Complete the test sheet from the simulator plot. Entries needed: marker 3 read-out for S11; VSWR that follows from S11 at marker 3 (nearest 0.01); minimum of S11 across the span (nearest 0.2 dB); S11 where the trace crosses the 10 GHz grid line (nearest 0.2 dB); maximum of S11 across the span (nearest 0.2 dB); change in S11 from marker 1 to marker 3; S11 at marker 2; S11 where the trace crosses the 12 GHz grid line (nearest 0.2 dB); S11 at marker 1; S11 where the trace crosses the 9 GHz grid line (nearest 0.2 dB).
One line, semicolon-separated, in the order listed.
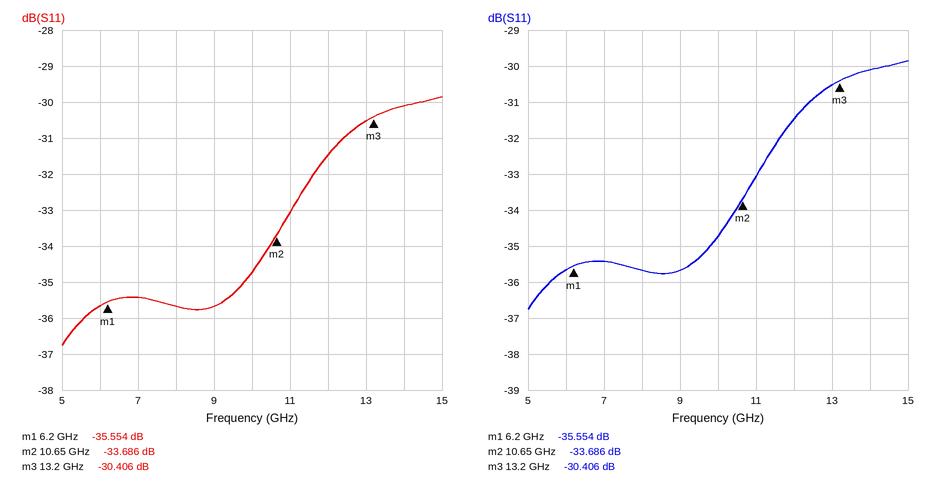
-30.406 dB; 1.06; -36.8 dB; -34.8 dB; -29.8 dB; 5.148 dB; -33.686 dB; -31.4 dB; -35.554 dB; -35.6 dB
